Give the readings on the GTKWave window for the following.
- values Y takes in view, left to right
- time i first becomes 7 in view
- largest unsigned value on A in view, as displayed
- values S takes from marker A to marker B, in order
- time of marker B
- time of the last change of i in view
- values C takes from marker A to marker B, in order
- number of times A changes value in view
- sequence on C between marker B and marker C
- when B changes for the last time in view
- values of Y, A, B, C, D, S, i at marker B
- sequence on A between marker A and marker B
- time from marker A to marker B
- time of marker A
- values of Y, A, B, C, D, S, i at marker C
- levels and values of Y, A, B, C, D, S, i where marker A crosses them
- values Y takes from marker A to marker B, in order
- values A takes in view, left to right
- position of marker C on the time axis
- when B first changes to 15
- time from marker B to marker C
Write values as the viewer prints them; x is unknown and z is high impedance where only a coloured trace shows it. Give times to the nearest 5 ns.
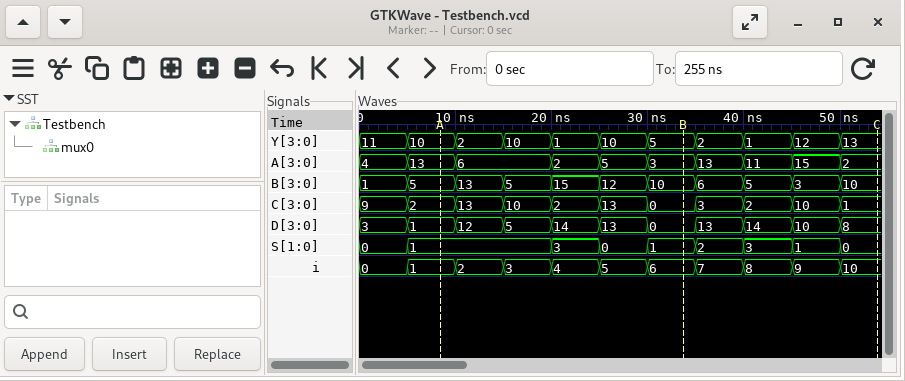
11, 10, 2, 10, 1, 10, 5, 2, 1, 12, 13
35 ns
15
1, 3, 0, 1
35 ns
50 ns
2, 13, 10, 2, 13, 0
9
0, 3, 2, 10, 1
50 ns
Y=5, A=3, B=10, C=0, D=0, S=1, i=6
13, 6, 2, 5, 3
25 ns
10 ns
Y=13, A=2, B=10, C=1, D=8, S=0, i=10
Y=10, A=13, B=5, C=2, D=1, S=1, i=1
10, 2, 10, 1, 10, 5
4, 13, 6, 2, 5, 3, 13, 11, 15, 2
55 ns
20 ns
20 ns
